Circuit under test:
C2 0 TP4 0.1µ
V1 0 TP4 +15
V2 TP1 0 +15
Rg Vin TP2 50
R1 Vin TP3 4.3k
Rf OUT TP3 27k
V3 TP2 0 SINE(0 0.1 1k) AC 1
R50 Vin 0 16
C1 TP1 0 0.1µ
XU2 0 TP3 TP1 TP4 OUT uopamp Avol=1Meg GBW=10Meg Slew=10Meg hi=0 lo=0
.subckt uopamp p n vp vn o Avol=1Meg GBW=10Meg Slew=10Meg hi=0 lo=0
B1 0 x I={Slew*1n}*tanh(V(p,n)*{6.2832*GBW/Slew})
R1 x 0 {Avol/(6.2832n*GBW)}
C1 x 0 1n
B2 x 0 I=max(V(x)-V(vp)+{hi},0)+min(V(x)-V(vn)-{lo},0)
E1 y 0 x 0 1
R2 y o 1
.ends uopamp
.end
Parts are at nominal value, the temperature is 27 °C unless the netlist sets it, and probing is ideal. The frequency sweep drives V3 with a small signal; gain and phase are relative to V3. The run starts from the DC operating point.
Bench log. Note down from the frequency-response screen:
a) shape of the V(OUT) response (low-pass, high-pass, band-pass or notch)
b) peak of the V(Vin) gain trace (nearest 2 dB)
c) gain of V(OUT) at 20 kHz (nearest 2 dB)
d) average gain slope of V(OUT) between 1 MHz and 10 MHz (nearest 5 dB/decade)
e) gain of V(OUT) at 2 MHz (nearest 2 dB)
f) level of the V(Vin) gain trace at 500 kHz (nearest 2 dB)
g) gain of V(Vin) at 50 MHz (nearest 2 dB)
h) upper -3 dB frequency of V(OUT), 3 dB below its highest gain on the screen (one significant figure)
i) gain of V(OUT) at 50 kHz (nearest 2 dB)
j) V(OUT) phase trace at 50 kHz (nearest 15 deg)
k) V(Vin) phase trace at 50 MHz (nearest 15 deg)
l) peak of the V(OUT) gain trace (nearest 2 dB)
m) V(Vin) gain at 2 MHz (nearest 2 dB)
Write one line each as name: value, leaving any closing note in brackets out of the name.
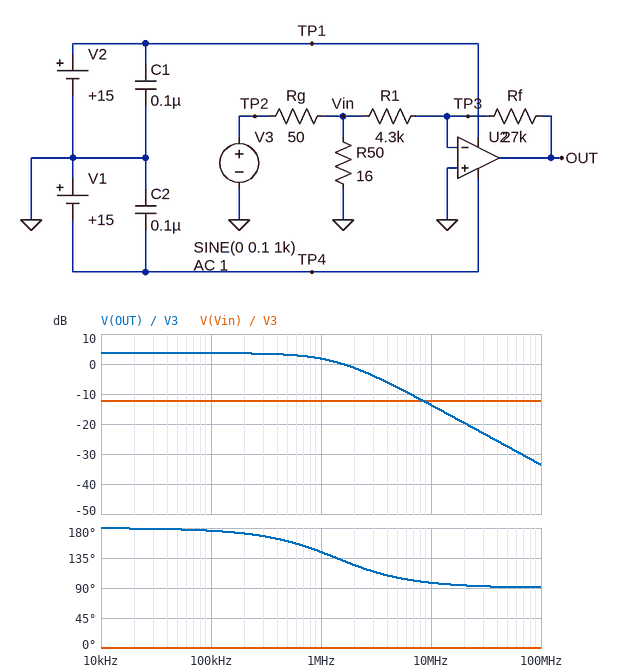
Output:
shape of the V(OUT) response: low-pass
peak of the V(Vin) gain trace: -12 dB
gain of V(OUT) at 20 kHz: 4 dB
average gain slope of V(OUT) between 1 MHz and 10 MHz: -15 dB/decade
gain of V(OUT) at 2 MHz: -2 dB
level of the V(Vin) gain trace at 500 kHz: -12 dB
gain of V(Vin) at 50 MHz: -12 dB
upper -3 dB frequency of V(OUT), 3 dB below its highest gain on the screen: 1 MHz
gain of V(OUT) at 50 kHz: 4 dB
V(OUT) phase trace at 50 kHz: 180 deg
V(Vin) phase trace at 50 MHz: 0 deg
peak of the V(OUT) gain trace: 4 dB
V(Vin) gain at 2 MHz: -12 dB
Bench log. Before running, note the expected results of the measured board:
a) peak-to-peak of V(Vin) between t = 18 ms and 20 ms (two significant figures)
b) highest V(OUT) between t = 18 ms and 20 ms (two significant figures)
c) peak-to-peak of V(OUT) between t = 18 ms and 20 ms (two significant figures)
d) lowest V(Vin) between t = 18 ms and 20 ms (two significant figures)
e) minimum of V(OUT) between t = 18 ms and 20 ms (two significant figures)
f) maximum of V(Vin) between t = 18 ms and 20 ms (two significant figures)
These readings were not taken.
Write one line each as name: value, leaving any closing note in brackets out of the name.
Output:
peak-to-peak of V(Vin) between t = 18 ms and 20 ms: 48 mV
highest V(OUT) between t = 18 ms and 20 ms: 150 mV
peak-to-peak of V(OUT) between t = 18 ms and 20 ms: 300 mV
lowest V(Vin) between t = 18 ms and 20 ms: -24 mV
minimum of V(OUT) between t = 18 ms and 20 ms: -150 mV
maximum of V(Vin) between t = 18 ms and 20 ms: 24 mV
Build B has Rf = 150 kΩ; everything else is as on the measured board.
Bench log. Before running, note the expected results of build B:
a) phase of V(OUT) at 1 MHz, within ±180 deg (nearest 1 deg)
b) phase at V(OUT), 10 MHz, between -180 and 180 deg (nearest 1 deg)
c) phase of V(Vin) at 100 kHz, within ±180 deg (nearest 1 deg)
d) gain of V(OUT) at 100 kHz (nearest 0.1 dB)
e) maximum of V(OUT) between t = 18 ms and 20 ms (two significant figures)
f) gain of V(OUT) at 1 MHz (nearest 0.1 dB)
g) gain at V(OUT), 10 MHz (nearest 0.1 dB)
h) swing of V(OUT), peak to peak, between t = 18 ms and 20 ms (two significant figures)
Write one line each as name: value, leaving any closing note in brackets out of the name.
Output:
phase of V(OUT) at 1 MHz, within ±180 deg: 106 deg
phase at V(OUT), 10 MHz, between -180 and 180 deg: 92 deg
phase of V(Vin) at 100 kHz, within ±180 deg: 0 deg
gain of V(OUT) at 100 kHz: 18.0 dB
maximum of V(OUT) between t = 18 ms and 20 ms: 840 mV
gain of V(OUT) at 1 MHz: 7.1 dB
gain at V(OUT), 10 MHz: -12.6 dB
swing of V(OUT), peak to peak, between t = 18 ms and 20 ms: 1.7 V
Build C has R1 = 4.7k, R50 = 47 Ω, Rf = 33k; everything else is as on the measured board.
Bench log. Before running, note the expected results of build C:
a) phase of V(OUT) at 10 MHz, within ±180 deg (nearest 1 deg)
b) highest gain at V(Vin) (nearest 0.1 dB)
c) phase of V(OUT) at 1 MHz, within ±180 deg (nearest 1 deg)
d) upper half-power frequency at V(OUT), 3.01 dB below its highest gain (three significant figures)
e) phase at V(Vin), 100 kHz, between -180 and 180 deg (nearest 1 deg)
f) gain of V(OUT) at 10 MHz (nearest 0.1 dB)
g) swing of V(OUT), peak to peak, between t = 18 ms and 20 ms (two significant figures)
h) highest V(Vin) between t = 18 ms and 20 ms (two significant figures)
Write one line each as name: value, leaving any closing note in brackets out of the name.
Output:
phase of V(OUT) at 10 MHz, within ±180 deg: 97 deg
highest gain at V(Vin): -6.3 dB
phase of V(OUT) at 1 MHz, within ±180 deg: 141 deg
upper half-power frequency at V(OUT), 3.01 dB below its highest gain: 1.25 MHz
phase at V(Vin), 100 kHz, between -180 and 180 deg: 0 deg
gain of V(OUT) at 10 MHz: -7.5 dB
swing of V(OUT), peak to peak, between t = 18 ms and 20 ms: 680 mV
highest V(Vin) between t = 18 ms and 20 ms: 48 mV
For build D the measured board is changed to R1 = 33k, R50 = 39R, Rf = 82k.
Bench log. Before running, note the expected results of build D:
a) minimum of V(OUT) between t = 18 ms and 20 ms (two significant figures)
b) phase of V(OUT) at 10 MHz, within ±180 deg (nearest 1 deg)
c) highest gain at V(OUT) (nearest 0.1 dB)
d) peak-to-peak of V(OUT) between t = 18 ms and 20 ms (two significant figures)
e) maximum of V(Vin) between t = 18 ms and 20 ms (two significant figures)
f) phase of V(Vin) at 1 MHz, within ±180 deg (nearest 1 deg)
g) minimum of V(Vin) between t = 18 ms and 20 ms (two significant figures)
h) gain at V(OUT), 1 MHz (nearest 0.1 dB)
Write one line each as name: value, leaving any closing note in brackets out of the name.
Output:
minimum of V(OUT) between t = 18 ms and 20 ms: -110 mV
phase of V(OUT) at 10 MHz, within ±180 deg: 106 deg
highest gain at V(OUT): 0.7 dB
peak-to-peak of V(OUT) between t = 18 ms and 20 ms: 220 mV
maximum of V(Vin) between t = 18 ms and 20 ms: 44 mV
phase of V(Vin) at 1 MHz, within ±180 deg: 0 deg
minimum of V(Vin) between t = 18 ms and 20 ms: -44 mV
gain at V(OUT), 1 MHz: 0.2 dB
